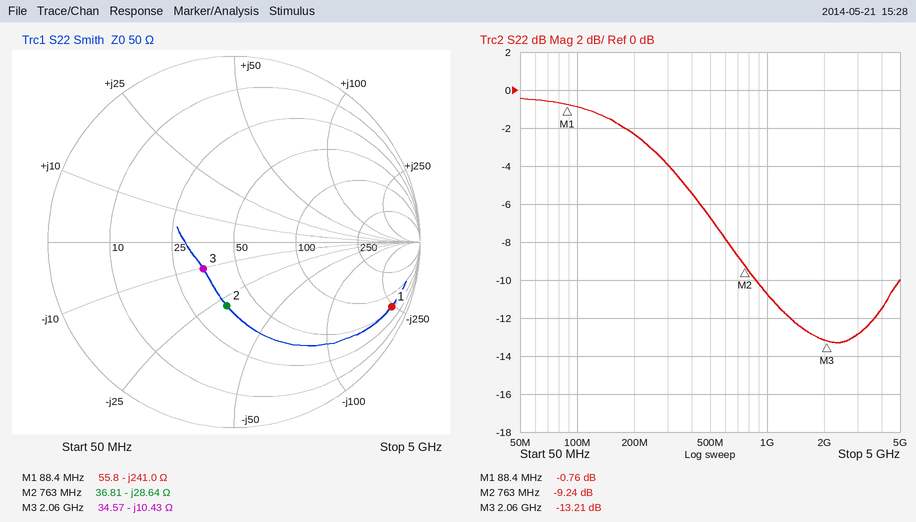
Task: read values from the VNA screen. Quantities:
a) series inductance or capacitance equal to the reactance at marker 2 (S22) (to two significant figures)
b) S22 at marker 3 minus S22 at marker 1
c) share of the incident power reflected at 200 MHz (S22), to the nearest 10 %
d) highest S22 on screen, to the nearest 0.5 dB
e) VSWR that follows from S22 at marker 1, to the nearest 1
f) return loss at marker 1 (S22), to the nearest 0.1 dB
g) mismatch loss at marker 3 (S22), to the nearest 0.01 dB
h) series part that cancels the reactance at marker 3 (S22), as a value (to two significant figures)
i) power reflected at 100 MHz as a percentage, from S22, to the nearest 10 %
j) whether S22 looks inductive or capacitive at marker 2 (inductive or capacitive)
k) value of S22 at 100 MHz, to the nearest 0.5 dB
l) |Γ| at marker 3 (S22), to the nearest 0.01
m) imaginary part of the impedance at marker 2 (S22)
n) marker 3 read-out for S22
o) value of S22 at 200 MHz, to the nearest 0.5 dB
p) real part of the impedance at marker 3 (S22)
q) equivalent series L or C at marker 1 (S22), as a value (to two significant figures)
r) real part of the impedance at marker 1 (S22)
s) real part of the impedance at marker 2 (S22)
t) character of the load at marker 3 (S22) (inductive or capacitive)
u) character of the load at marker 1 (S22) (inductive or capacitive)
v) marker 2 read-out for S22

7.3 pF
-12.45 dB
60 %
-0.5 dB
23
0.8 dB
0.21 dB
810 pH
80 %
capacitive
-1.0 dB
0.22
-28.64 Ω
-13.21 dB
-2.5 dB
34.57 Ω
7.5 pF
55.8 Ω
36.81 Ω
capacitive
capacitive
-9.24 dB
